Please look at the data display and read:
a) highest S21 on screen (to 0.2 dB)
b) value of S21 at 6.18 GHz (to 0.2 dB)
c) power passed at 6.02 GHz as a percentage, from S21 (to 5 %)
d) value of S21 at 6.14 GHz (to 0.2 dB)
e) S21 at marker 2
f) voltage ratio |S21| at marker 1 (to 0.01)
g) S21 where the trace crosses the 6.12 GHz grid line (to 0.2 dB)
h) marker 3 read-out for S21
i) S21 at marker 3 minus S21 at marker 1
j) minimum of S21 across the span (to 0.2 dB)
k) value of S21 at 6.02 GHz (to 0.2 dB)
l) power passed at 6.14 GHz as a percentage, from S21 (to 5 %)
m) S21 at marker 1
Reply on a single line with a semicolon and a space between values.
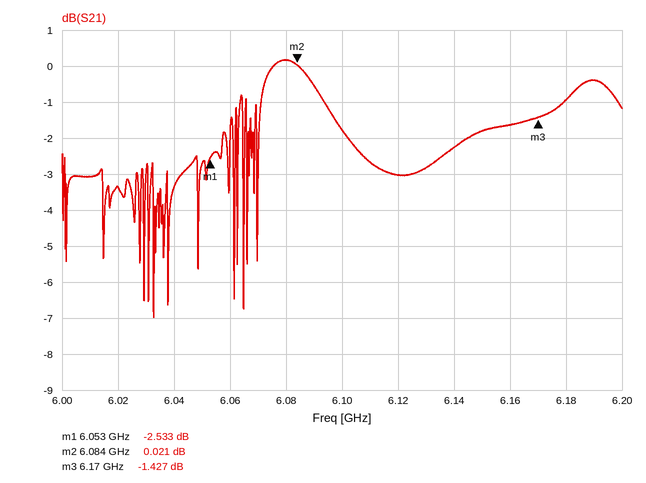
0.2 dB; -1.0 dB; 45 %; -2.2 dB; 0.021 dB; 0.75; -3.0 dB; -1.427 dB; 1.106 dB; -7.0 dB; -3.4 dB; 60 %; -2.533 dB
